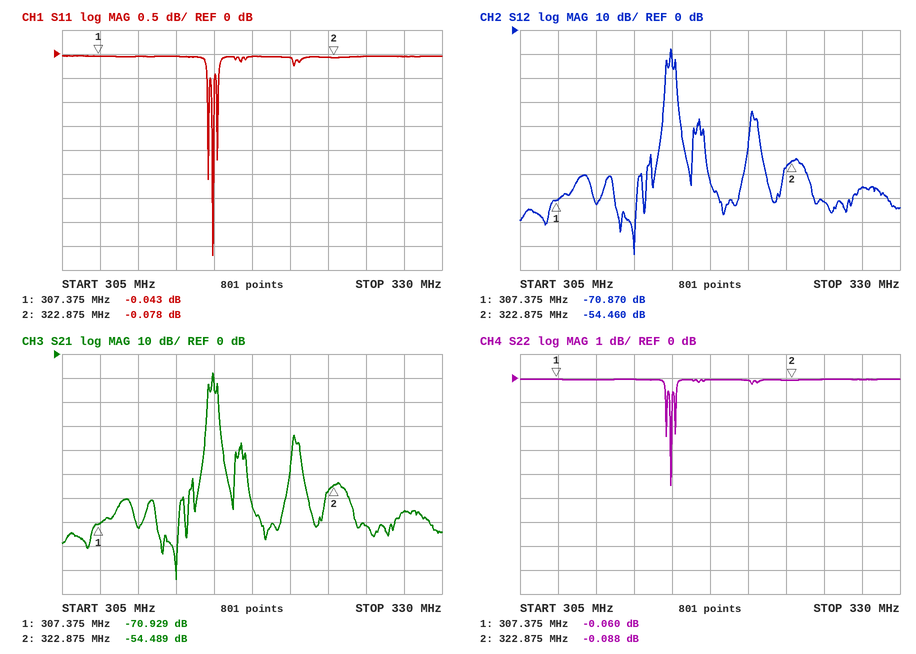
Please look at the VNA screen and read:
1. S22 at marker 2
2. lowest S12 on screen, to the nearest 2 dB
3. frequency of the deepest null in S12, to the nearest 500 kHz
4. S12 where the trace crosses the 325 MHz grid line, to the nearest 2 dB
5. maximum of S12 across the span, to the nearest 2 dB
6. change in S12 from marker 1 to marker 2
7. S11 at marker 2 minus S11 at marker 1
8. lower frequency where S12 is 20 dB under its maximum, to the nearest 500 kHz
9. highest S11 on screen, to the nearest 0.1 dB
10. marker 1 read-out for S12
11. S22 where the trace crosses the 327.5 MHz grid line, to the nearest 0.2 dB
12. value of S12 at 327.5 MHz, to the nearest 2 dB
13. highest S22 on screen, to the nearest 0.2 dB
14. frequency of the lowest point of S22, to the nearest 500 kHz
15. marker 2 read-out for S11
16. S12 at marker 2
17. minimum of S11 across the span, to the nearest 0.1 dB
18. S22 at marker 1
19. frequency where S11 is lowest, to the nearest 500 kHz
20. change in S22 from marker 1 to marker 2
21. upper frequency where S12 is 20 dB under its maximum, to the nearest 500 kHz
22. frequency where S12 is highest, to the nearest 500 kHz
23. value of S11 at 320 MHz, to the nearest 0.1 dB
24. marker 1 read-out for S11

-0.088 dB
-94 dB
312.5 MHz
-72 dB
-8 dB
16.410 dB
-0.035 dB
314.5 MHz
0.0 dB
-70.870 dB
0.0 dB
-66 dB
0.0 dB
315.0 MHz
-0.078 dB
-54.460 dB
-4.2 dB
-0.060 dB
315.0 MHz
-0.028 dB
315.5 MHz
315.0 MHz
-0.1 dB
-0.043 dB
